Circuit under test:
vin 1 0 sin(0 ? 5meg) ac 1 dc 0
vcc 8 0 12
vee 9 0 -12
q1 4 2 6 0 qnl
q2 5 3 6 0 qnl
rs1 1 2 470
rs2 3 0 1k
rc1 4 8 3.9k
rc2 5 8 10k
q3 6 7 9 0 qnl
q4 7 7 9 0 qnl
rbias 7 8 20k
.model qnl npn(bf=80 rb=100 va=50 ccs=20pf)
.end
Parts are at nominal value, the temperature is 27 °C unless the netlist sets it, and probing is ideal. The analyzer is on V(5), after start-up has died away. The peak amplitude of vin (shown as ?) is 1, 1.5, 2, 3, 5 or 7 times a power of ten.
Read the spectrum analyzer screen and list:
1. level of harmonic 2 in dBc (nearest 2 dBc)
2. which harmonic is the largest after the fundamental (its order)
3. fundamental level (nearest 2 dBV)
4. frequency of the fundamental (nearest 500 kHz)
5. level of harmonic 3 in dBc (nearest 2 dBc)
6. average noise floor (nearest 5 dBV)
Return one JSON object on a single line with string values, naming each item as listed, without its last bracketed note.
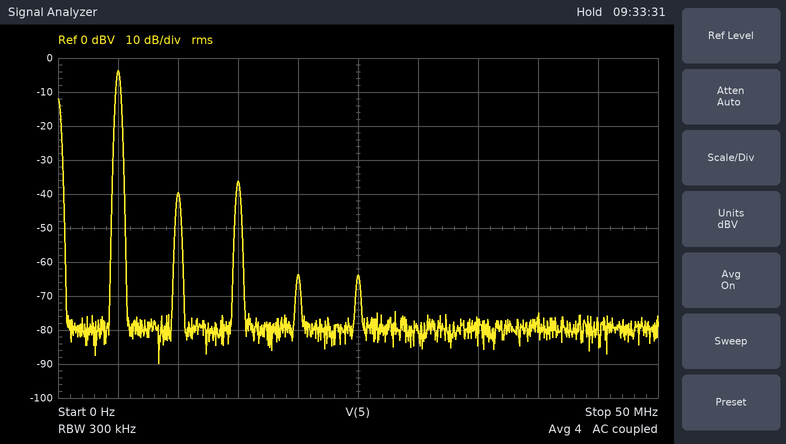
{"level of harmonic 2 in dBc": "-36 dBc", "which harmonic is the largest after the fundamental": "3", "fundamental level": "-4 dBV", "frequency of the fundamental": "5.0 MHz", "level of harmonic 3 in dBc": "-32 dBc", "average noise floor": "-80 dBV"}
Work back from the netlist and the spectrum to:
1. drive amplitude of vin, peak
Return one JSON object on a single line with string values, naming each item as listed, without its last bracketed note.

{"drive amplitude of vin, peak": "70 mV"}
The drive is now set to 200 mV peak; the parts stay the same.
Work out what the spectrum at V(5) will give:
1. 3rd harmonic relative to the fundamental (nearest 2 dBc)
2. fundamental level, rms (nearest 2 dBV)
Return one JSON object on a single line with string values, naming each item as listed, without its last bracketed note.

{"3rd harmonic relative to the fundamental": "-22 dBc", "fundamental level, rms": "0 dBV"}
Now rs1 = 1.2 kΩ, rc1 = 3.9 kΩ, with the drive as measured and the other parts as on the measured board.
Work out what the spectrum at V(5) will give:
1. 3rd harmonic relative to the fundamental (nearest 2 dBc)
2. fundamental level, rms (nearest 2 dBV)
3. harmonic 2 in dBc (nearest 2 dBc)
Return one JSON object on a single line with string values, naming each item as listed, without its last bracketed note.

{"3rd harmonic relative to the fundamental": "-34 dBc", "fundamental level, rms": "-4 dBV", "harmonic 2 in dBc": "-52 dBc"}
